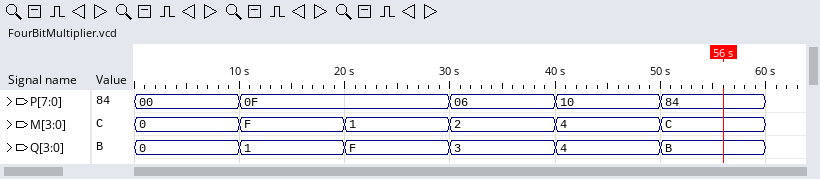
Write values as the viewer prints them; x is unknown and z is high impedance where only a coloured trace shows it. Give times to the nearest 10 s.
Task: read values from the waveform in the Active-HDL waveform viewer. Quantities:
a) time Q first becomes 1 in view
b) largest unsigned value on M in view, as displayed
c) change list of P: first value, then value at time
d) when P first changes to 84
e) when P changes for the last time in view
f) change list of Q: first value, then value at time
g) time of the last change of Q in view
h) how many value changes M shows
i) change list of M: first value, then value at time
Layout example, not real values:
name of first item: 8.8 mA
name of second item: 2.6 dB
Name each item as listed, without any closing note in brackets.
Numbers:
time Q first becomes 1 in view: 10 s
largest unsigned value on M in view, as displayed: F
change list of P: first value, then value at time: 00, 0F at 10 s, 06 at 30 s, 10 at 40 s, 84 at 50 s
when P first changes to 84: 50 s
when P changes for the last time in view: 50 s
change list of Q: first value, then value at time: 0, 1 at 10 s, F at 20 s, 3 at 30 s, 4 at 40 s, B at 50 s
time of the last change of Q in view: 50 s
how many value changes M shows: 5
change list of M: first value, then value at time: 0, F at 10 s, 1 at 20 s, 2 at 30 s, 4 at 40 s, C at 50 s
